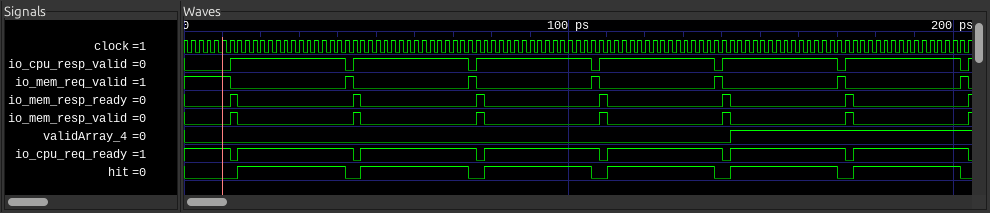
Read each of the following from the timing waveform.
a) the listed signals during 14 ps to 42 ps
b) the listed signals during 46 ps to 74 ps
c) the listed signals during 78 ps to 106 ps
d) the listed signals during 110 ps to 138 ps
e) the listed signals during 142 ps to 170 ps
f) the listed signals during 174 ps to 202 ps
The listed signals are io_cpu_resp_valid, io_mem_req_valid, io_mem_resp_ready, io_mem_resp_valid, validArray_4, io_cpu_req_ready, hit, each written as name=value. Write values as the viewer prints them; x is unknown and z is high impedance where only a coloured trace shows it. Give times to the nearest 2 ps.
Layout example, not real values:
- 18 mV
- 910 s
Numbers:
- io_cpu_resp_valid=1, io_mem_req_valid=0, io_mem_resp_ready=0, io_mem_resp_valid=0, validArray_4=0, io_cpu_req_ready=1, hit=1
- io_cpu_resp_valid=1, io_mem_req_valid=0, io_mem_resp_ready=0, io_mem_resp_valid=0, validArray_4=0, io_cpu_req_ready=1, hit=1
- io_cpu_resp_valid=1, io_mem_req_valid=0, io_mem_resp_ready=0, io_mem_resp_valid=0, validArray_4=0, io_cpu_req_ready=1, hit=1
- io_cpu_resp_valid=1, io_mem_req_valid=0, io_mem_resp_ready=0, io_mem_resp_valid=0, validArray_4=0, io_cpu_req_ready=1, hit=1
- io_cpu_resp_valid=1, io_mem_req_valid=0, io_mem_resp_ready=0, io_mem_resp_valid=0, validArray_4=1, io_cpu_req_ready=1, hit=1
- io_cpu_resp_valid=1, io_mem_req_valid=0, io_mem_resp_ready=0, io_mem_resp_valid=0, validArray_4=1, io_cpu_req_ready=1, hit=1
